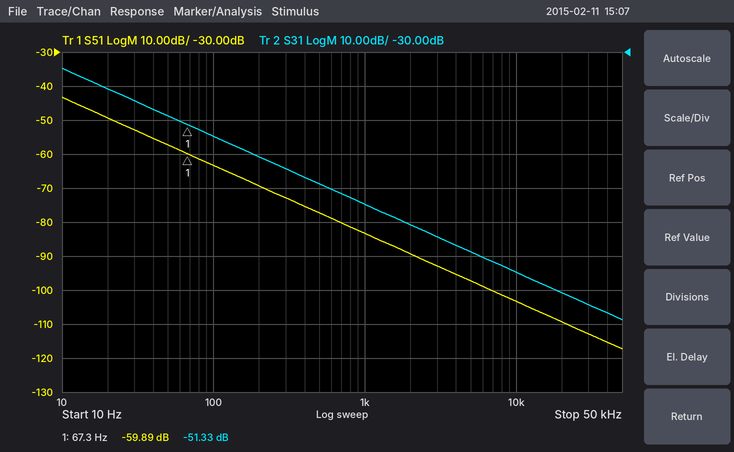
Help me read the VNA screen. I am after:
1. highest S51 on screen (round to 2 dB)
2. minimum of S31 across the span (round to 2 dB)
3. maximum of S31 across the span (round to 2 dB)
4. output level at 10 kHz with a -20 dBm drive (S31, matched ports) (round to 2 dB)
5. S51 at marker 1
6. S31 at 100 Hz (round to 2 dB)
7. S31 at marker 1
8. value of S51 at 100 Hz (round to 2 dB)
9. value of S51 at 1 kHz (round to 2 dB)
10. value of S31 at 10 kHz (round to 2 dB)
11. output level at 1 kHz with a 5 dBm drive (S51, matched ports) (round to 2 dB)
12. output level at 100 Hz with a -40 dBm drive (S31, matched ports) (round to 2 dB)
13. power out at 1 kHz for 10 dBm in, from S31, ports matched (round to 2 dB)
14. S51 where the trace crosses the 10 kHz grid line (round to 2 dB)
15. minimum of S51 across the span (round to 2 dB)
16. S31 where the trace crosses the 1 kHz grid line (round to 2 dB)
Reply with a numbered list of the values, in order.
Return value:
1. -44 dB
2. -108 dB
3. -34 dB
4. -114 dBm
5. -59.89 dB
6. -54 dB
7. -51.33 dB
8. -64 dB
9. -84 dB
10. -94 dB
11. -78 dBm
12. -94 dBm
13. -64 dBm
14. -104 dB
15. -118 dB
16. -74 dB
